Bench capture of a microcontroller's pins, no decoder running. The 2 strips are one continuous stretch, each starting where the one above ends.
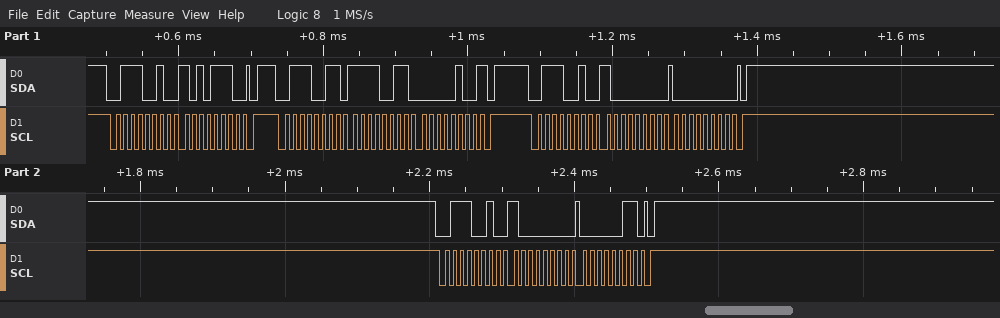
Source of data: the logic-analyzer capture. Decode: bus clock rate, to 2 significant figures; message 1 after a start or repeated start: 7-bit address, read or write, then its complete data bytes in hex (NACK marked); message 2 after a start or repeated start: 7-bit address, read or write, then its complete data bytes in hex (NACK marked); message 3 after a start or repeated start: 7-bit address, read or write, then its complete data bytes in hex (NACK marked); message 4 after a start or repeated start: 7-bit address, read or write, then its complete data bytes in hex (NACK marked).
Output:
100 kHz
0x39 write: AE
0x39 read: F3 04 NACK
0x39 write: 80 00
0x39 write: 80 03
